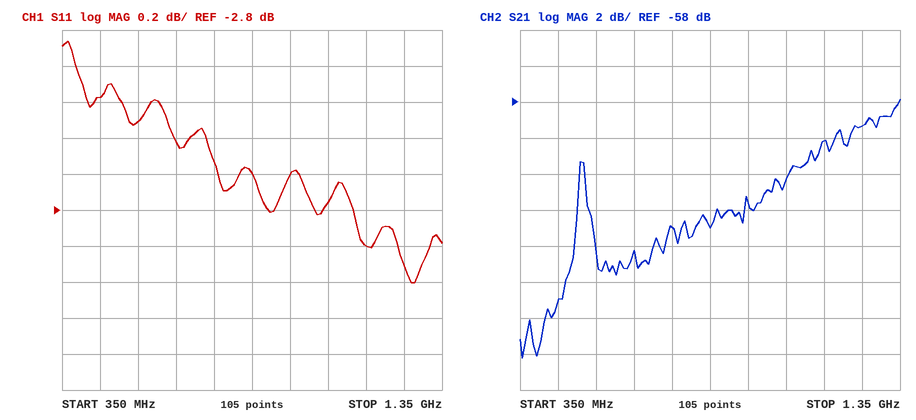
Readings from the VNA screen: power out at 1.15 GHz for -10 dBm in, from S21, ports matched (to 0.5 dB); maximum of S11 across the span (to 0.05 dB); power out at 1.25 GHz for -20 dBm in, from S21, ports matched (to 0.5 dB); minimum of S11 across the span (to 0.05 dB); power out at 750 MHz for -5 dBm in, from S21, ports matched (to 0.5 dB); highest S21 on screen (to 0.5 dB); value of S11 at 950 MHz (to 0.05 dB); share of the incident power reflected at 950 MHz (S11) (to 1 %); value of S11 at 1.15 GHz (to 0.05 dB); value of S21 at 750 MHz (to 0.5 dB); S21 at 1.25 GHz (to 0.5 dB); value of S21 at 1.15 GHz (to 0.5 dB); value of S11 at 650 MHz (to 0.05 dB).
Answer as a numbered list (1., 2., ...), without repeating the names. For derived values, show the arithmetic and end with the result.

1. -10 dBm + (-60.0 dB) = -70.0 dBm
2. -1.85 dB
3. -20 dBm + (-59.5 dB) = -79.5 dBm
4. -3.20 dB
5. -5 dBm + (-65.0 dB) = -70.0 dBm
6. -58.0 dB
7. -2.60 dB
8. 10^(-2.6/10) ≈ 55 %
9. -3.00 dB
10. -65.0 dB
11. -59.5 dB
12. -60.0 dB
13. -2.40 dB
